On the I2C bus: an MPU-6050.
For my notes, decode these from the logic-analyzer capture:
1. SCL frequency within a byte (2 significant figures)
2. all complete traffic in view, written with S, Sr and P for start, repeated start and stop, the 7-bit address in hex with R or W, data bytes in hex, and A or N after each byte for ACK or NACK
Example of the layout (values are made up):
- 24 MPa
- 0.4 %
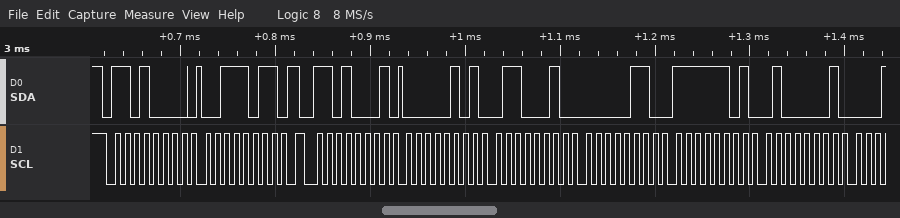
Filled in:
- 100 kHz
- S 68W A 3B A Sr 68R A 05 A 62 A 06 A FD A 41 A
